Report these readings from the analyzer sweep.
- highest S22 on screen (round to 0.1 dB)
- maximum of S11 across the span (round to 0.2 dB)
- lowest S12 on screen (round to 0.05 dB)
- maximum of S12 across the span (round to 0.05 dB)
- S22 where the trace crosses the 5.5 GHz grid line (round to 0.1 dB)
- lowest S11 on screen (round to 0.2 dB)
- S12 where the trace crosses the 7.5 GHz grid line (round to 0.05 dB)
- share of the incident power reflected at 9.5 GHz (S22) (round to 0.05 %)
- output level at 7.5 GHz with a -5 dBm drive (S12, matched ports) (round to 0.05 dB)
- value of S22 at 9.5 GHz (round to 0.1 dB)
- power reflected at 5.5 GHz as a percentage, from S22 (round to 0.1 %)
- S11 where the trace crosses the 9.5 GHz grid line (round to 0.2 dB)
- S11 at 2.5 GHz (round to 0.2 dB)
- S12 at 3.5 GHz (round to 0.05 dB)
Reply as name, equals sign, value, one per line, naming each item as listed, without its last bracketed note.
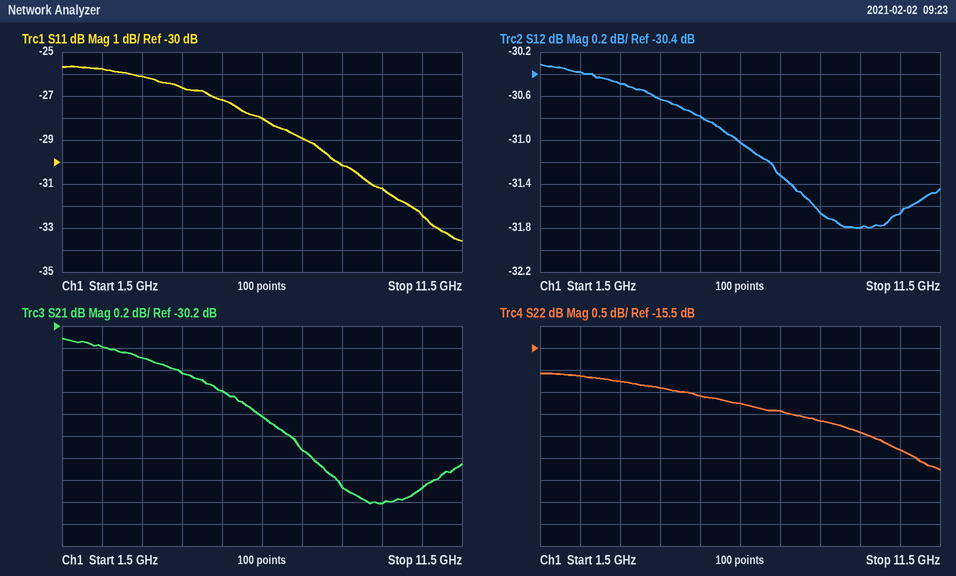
highest S22 on screen = -16.1 dB
maximum of S11 across the span = -25.6 dB
lowest S12 on screen = -31.80 dB
maximum of S12 across the span = -30.30 dB
S22 where the trace crosses the 5.5 GHz grid line = -16.6 dB
lowest S11 on screen = -33.6 dB
S12 where the trace crosses the 7.5 GHz grid line = -31.30 dB
share of the incident power reflected at 9.5 GHz (S22) = 1.80 %
output level at 7.5 GHz with a -5 dBm drive (S12, matched ports) = -36.30 dBm
value of S22 at 9.5 GHz = -17.4 dB
power reflected at 5.5 GHz as a percentage, from S22 = 2.2 %
S11 where the trace crosses the 9.5 GHz grid line = -31.2 dB
S11 at 2.5 GHz = -25.8 dB
S12 at 3.5 GHz = -30.50 dB
